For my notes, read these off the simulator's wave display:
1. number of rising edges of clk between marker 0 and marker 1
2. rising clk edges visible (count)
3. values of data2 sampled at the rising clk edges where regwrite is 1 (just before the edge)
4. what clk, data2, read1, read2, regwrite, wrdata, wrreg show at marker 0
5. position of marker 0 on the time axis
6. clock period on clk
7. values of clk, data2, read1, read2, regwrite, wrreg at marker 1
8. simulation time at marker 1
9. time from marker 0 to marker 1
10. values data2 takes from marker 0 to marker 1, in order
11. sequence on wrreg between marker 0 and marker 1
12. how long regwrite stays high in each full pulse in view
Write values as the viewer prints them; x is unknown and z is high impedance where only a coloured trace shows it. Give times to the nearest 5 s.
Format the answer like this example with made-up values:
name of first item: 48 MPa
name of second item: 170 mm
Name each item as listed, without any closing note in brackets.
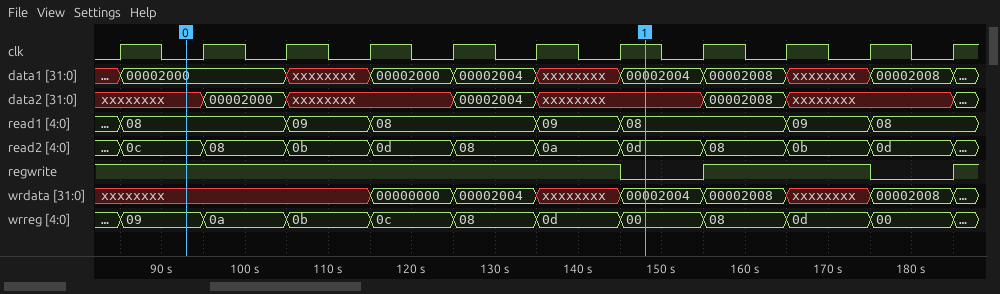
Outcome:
number of rising edges of clk between marker 0 and marker 1: 6
rising clk edges visible: 11
values of data2 sampled at the rising clk edges where regwrite is 1: xxxxxxxx, xxxxxxxx, 00002000, xxxxxxxx, xxxxxxxx, 00002004, xxxxxxxx, 00002008, xxxxxxxx
what clk, data2, read1, read2, regwrite, wrdata, wrreg show at marker 0: clk=0, data2=xxxxxxxx, read1=08, read2=0c, regwrite=1, wrdata=xxxxxxxx, wrreg=09
position of marker 0 on the time axis: 95 s
clock period on clk: 10 s
values of clk, data2, read1, read2, regwrite, wrreg at marker 1: clk=1, data2=xxxxxxxx, read1=08, read2=0d, regwrite=0, wrreg=00
simulation time at marker 1: 150 s
time from marker 0 to marker 1: 55 s
values data2 takes from marker 0 to marker 1, in order: xxxxxxxx, 00002000, xxxxxxxx, 00002004, xxxxxxxx
sequence on wrreg between marker 0 and marker 1: 09, 0a, 0b, 0c, 08, 0d, 00
how long regwrite stays high in each full pulse in view: 20 s
